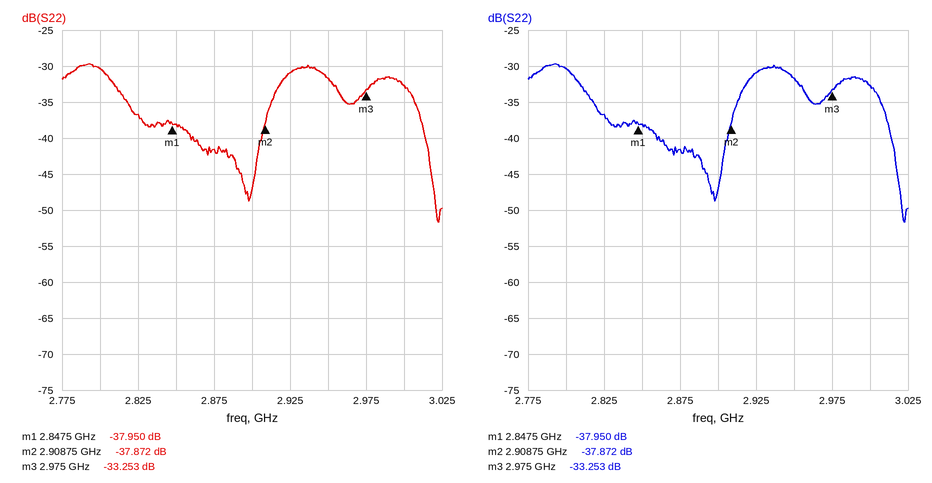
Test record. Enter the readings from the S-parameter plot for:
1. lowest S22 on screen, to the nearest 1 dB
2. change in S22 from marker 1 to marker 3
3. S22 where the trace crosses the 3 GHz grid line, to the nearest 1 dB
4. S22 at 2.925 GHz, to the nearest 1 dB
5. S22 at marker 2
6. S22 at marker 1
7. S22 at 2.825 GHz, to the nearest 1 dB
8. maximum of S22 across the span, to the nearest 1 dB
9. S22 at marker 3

-52 dB
4.697 dB
-33 dB
-31 dB
-37.872 dB
-37.950 dB
-37 dB
-30 dB
-33.253 dB
